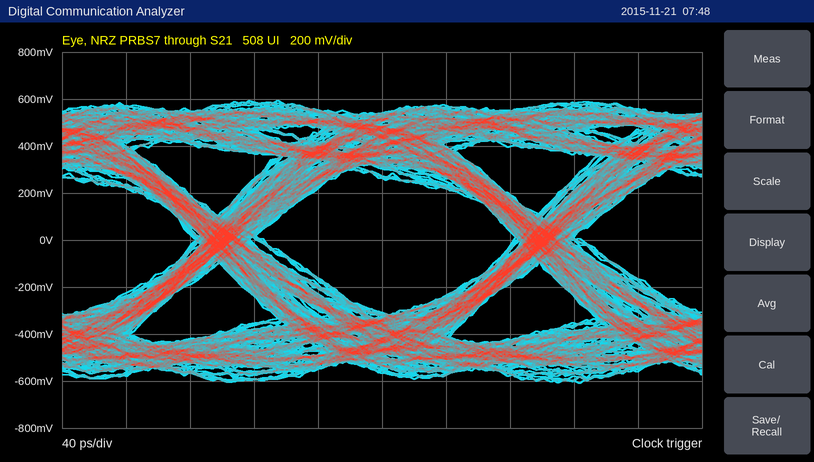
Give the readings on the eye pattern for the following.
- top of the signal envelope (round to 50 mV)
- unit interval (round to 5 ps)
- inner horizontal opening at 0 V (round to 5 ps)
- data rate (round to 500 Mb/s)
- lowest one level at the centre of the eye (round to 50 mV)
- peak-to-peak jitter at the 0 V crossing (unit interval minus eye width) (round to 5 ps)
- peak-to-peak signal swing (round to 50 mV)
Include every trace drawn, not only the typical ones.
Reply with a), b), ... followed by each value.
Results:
a) 600 mV
b) 200 ps
c) 155 ps
d) 5.0 Gb/s
e) 250 mV
f) 45 ps
g) 1.20 V
